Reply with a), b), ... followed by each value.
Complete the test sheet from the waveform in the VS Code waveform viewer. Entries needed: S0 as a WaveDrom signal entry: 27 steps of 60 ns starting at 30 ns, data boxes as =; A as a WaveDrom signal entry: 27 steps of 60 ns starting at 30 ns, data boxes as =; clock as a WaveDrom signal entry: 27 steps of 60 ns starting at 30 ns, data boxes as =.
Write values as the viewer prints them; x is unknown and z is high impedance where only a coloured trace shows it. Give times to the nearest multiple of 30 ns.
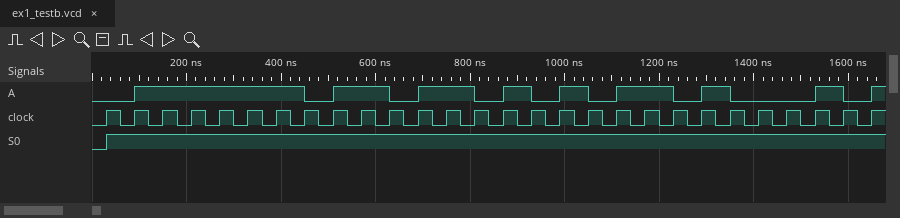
a) {name: 'S0', wave: '1..........................'}
b) {name: 'A', wave: '01.....01.01.010101.010..10'}
c) {name: 'clock', wave: 'p..........................'}
